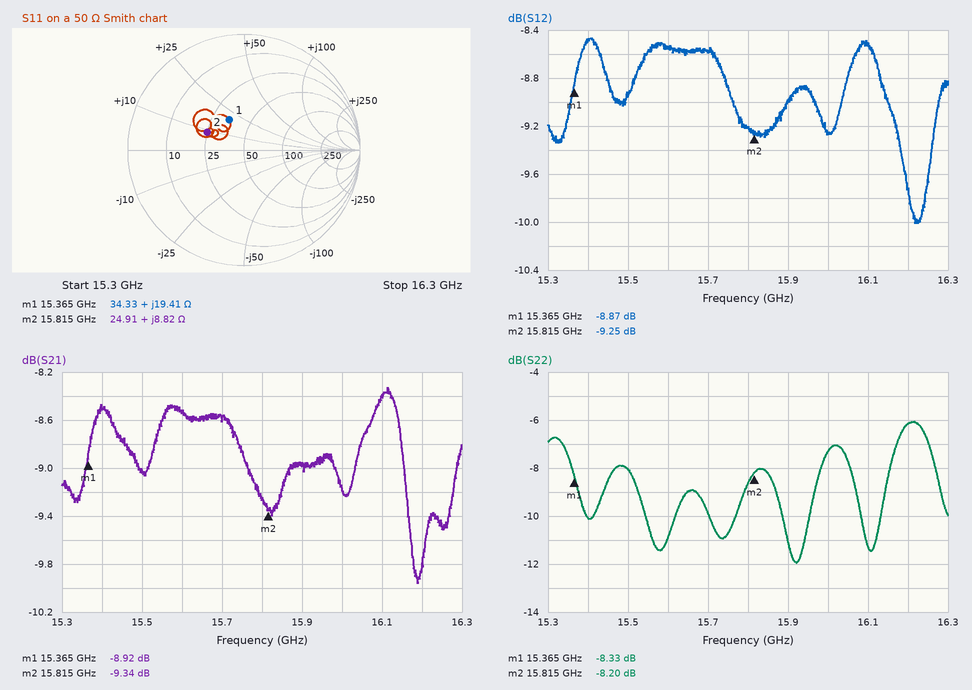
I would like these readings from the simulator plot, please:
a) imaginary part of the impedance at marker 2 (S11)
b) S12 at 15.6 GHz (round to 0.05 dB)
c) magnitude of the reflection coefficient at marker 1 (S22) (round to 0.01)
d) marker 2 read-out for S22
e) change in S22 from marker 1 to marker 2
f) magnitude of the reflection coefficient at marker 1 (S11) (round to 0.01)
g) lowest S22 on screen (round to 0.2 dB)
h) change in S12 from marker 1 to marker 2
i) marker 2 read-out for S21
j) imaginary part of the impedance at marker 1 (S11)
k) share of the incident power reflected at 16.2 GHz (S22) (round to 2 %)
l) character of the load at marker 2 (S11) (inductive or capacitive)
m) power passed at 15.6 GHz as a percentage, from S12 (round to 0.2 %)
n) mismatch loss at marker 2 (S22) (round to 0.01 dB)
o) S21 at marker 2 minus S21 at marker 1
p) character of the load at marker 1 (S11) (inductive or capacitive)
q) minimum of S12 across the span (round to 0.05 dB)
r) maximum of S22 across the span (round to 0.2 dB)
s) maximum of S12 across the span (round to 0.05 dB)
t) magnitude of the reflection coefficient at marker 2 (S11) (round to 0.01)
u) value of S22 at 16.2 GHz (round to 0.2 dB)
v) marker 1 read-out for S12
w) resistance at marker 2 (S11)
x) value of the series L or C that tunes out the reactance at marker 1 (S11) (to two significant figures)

+8.82 Ω
-8.55 dB
0.38
-8.20 dB
0.13 dB
0.29
-12.0 dB
-0.38 dB
-9.34 dB
+19.41 Ω
24 %
inductive
14.0 %
0.71 dB
-0.42 dB
inductive
-10.00 dB
-6.0 dB
-8.45 dB
0.35
-6.2 dB
-8.87 dB
24.91 Ω
530 fF
